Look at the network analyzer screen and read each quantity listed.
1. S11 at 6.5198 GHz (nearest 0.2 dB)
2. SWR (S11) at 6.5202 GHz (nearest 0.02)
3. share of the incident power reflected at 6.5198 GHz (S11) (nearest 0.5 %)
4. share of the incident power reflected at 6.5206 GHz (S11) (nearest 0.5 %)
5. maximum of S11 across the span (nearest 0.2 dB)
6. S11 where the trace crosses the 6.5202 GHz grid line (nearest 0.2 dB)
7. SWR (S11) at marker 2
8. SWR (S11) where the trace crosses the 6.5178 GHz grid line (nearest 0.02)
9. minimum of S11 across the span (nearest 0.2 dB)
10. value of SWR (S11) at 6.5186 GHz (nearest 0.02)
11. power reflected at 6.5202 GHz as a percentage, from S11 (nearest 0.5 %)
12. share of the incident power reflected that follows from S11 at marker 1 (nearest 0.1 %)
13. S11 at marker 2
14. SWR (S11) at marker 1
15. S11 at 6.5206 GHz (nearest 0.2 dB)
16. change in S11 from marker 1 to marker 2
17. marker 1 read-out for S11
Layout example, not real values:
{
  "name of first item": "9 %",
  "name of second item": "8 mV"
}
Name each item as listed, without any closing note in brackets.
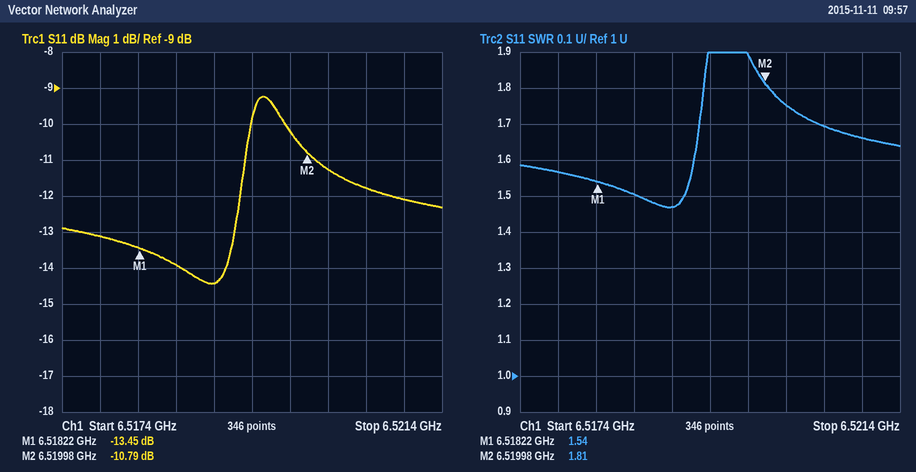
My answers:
{
  "S11 at 6.5198 GHz": "-10.2 dB",
  "SWR (S11) at 6.5202 GHz": "1.76",
  "share of the incident power reflected at 6.5198 GHz (S11)": "9.5 %",
  "share of the incident power reflected at 6.5206 GHz (S11)": "6.5 %",
  "maximum of S11 across the span": "-9.2 dB",
  "S11 where the trace crosses the 6.5202 GHz grid line": "-11.2 dB",
  "SWR (S11) at marker 2": "1.81",
  "SWR (S11) where the trace crosses the 6.5178 GHz grid line": "1.56",
  "minimum of S11 across the span": "-14.4 dB",
  "value of SWR (S11) at 6.5186 GHz": "1.50",
  "power reflected at 6.5202 GHz as a percentage, from S11": "7.5 %",
  "share of the incident power reflected that follows from S11 at marker 1": "4.5 %",
  "S11 at marker 2": "-10.79 dB",
  "SWR (S11) at marker 1": "1.54",
  "S11 at 6.5206 GHz": "-11.8 dB",
  "change in S11 from marker 1 to marker 2": "2.66 dB",
  "marker 1 read-out for S11": "-13.45 dB"
}
